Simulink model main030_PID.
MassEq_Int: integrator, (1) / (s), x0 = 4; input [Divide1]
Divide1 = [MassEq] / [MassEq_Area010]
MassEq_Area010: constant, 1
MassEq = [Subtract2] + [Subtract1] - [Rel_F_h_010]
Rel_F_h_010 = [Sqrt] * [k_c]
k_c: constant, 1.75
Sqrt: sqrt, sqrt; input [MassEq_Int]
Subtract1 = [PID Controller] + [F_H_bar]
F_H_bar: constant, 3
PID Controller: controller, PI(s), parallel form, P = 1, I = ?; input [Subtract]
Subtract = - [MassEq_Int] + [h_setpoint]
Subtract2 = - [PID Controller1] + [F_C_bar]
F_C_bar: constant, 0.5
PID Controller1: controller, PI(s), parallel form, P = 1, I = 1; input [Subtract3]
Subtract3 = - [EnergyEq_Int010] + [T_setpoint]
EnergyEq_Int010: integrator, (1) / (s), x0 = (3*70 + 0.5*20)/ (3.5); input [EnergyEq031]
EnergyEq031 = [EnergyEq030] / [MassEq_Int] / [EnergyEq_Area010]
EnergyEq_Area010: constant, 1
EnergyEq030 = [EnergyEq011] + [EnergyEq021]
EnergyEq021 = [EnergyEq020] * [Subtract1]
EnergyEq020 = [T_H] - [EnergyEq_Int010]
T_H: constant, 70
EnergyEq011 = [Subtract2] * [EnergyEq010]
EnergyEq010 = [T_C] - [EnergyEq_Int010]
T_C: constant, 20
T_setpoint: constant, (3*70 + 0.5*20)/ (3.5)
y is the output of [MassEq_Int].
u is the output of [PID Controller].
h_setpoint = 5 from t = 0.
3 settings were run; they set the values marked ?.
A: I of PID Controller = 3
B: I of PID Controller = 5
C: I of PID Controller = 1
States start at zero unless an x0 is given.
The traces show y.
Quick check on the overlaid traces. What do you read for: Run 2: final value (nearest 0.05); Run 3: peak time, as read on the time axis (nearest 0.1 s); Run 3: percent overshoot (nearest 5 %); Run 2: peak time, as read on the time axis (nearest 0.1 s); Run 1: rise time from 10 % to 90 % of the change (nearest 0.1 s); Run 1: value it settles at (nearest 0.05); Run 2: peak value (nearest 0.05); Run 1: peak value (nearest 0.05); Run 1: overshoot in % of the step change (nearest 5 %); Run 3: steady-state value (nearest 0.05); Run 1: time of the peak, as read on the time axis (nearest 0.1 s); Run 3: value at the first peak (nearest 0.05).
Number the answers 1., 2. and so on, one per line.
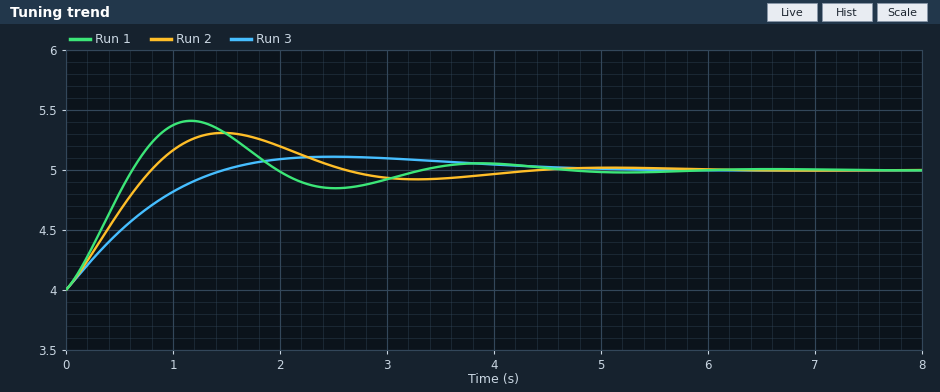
1. 5.00
2. 2.5 s
3. 10 %
4. 1.5 s
5. 0.5 s
6. 5.00
7. 5.30
8. 5.40
9. 40 %
10. 5.00
11. 1.2 s
12. 5.10
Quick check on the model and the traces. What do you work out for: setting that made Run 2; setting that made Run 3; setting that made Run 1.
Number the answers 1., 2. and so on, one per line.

1. A
2. C
3. B
